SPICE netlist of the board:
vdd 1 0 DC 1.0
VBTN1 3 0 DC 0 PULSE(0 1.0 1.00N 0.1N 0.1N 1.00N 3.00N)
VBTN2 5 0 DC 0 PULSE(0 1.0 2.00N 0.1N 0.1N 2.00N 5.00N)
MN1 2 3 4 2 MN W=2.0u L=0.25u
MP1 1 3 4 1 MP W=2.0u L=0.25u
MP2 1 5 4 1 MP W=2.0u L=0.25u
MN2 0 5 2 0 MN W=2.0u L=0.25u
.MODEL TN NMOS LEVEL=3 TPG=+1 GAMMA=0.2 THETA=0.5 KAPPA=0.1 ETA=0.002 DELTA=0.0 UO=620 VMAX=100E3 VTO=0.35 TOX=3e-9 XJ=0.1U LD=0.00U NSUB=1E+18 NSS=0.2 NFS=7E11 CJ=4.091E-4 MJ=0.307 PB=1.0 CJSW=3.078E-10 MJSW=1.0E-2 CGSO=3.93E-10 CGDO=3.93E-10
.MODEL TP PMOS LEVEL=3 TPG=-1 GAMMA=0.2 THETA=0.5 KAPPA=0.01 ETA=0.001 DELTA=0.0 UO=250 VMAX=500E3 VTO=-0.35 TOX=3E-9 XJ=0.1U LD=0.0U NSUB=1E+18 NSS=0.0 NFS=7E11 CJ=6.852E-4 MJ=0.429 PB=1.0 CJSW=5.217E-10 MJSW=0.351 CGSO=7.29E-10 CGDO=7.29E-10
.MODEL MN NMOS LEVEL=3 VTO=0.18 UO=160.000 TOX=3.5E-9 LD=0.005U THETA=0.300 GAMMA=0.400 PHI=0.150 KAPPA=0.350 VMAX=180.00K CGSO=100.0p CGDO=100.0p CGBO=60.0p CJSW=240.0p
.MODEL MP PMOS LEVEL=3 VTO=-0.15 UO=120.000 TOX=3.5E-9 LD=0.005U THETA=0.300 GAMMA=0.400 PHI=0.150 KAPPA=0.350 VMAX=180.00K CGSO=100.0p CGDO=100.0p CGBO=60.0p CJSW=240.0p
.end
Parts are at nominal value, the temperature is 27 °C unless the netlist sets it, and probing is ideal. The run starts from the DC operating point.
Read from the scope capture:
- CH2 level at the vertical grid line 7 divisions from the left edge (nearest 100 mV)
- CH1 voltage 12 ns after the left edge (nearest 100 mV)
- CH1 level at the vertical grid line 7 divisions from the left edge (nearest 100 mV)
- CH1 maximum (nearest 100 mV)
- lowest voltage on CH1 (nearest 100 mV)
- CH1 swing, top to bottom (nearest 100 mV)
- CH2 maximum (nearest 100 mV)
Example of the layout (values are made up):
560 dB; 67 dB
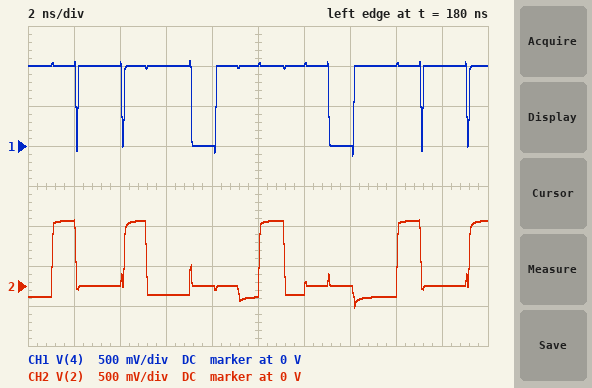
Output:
0 V; 1.0 V; 0 V; 1.1 V; -100 mV; 1.2 V; 800 mV
